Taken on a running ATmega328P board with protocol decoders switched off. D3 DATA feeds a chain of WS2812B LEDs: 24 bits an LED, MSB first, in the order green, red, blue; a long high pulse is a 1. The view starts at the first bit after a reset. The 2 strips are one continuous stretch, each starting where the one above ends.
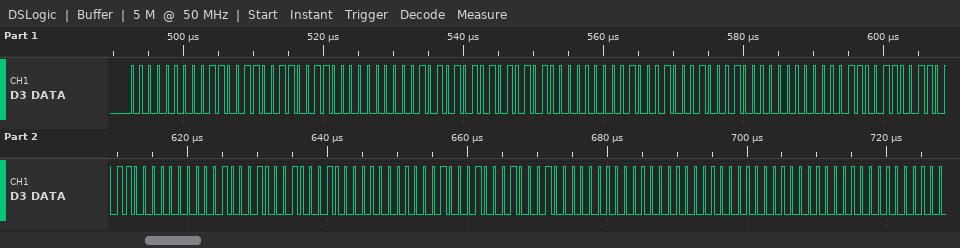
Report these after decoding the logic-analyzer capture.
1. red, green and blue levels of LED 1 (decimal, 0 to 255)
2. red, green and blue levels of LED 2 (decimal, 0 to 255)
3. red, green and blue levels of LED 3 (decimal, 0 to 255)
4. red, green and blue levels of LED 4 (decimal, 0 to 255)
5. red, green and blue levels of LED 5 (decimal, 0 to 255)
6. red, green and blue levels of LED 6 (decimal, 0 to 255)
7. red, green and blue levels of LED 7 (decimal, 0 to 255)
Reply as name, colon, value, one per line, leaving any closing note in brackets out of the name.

red, green and blue levels of LED 1: 102, 0, 102
red, green and blue levels of LED 2: 85, 0, 85
red, green and blue levels of LED 3: 68, 0, 68
red, green and blue levels of LED 4: 51, 0, 51
red, green and blue levels of LED 5: 34, 0, 34
red, green and blue levels of LED 6: 17, 0, 17
red, green and blue levels of LED 7: 0, 0, 0
